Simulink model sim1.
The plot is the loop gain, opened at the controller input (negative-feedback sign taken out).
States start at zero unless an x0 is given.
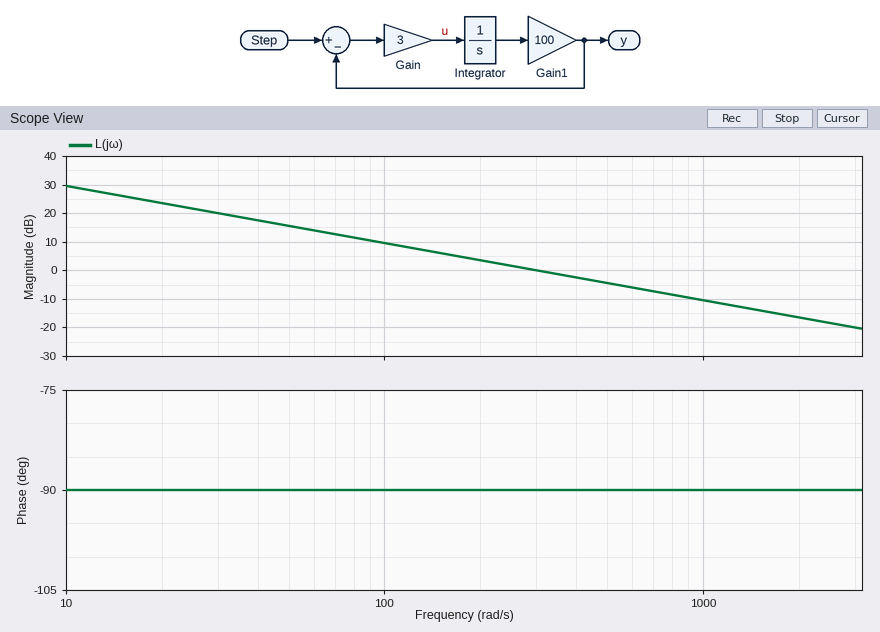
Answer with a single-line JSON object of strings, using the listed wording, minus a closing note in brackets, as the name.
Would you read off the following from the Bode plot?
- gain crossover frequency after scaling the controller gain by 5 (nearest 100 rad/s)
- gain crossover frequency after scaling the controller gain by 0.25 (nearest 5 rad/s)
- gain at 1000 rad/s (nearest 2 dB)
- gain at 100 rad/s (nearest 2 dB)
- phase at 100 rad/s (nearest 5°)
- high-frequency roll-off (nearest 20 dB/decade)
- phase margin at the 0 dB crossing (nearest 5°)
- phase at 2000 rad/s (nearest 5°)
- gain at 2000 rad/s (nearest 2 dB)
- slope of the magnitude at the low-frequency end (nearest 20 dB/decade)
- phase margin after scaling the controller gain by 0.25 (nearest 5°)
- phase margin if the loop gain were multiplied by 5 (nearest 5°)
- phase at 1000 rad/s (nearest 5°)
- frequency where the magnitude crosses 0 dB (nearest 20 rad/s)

{"gain crossover frequency after scaling the controller gain by 5": "1500 rad/s", "gain crossover frequency after scaling the controller gain by 0.25": "75 rad/s", "gain at 1000 rad/s": "-10 dB", "gain at 100 rad/s": "10 dB", "phase at 100 rad/s": "-90°", "high-frequency roll-off": "-20 dB/decade", "phase margin at the 0 dB crossing": "90°", "phase at 2000 rad/s": "-90°", "gain at 2000 rad/s": "-16 dB", "slope of the magnitude at the low-frequency end": "-20 dB/decade", "phase margin after scaling the controller gain by 0.25": "90°", "phase margin if the loop gain were multiplied by 5": "90°", "phase at 1000 rad/s": "-90°", "frequency where the magnitude crosses 0 dB": "300 rad/s"}
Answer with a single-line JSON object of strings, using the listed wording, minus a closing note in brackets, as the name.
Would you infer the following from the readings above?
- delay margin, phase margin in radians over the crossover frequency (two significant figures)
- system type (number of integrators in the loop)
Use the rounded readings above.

{"delay margin, phase margin in radians over the crossover frequency": "0.0052 s", "system type": "1"}
